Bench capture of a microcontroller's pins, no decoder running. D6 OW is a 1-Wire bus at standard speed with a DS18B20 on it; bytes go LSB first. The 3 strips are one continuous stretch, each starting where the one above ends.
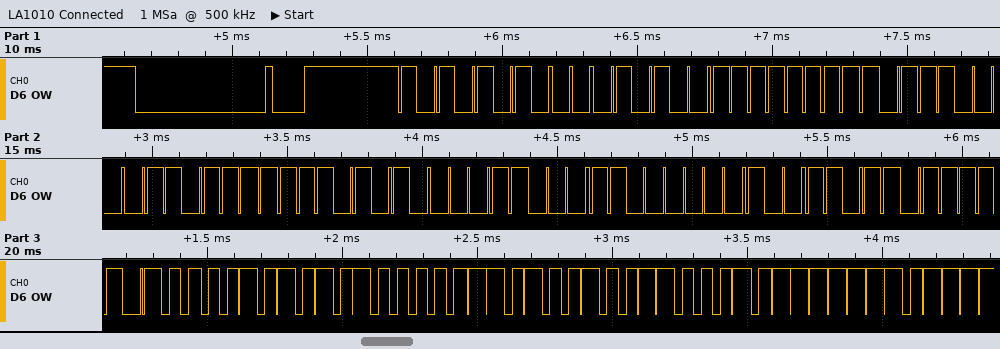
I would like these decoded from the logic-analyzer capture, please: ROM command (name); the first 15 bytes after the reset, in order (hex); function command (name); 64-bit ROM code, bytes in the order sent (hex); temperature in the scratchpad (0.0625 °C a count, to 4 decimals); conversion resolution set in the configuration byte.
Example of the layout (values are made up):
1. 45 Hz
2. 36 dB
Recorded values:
1. Match ROM
2. 55 28 FF 1D F6 57 18 03 D9 BE 50 05 4B 46 7F
3. Read Scratchpad
4. 28 FF 1D F6 57 18 03 D9
5. 85.0000 °C
6. 12 bits
